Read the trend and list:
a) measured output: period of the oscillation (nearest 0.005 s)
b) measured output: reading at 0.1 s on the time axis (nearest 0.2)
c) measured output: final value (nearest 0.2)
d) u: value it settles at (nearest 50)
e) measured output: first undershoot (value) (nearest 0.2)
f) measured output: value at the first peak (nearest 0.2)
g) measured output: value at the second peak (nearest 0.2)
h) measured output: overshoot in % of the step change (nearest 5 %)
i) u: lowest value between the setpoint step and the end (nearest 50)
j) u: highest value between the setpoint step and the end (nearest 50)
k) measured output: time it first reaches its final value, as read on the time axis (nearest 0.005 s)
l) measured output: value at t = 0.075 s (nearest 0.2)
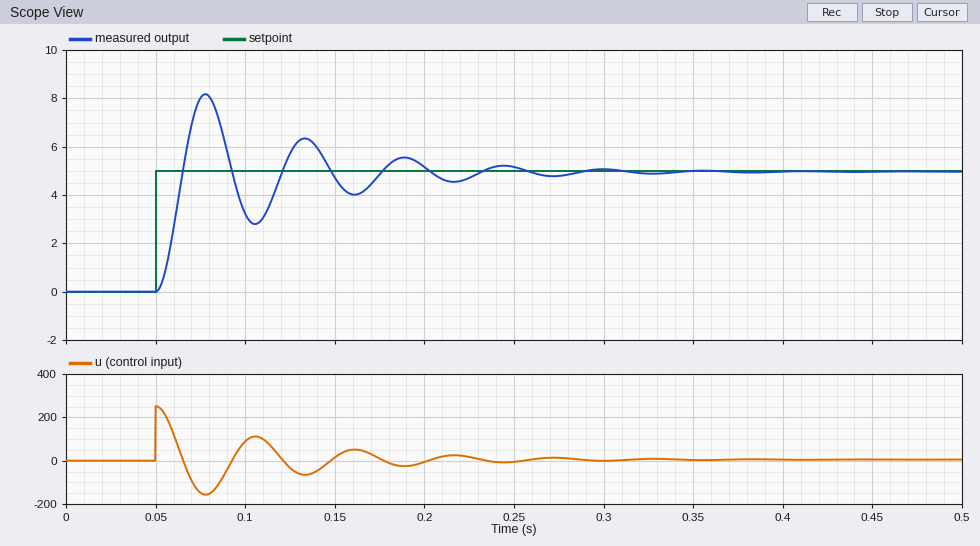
0.055 s
3.2
5.0
0
2.8
8.2
6.4
65 %
-150
250
0.065 s
8.0
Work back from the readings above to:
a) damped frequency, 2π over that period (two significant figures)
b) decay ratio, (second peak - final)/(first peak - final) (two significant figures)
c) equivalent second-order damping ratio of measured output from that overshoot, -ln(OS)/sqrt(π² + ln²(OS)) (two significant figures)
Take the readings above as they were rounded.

110 rad/s
0.44
0.14
